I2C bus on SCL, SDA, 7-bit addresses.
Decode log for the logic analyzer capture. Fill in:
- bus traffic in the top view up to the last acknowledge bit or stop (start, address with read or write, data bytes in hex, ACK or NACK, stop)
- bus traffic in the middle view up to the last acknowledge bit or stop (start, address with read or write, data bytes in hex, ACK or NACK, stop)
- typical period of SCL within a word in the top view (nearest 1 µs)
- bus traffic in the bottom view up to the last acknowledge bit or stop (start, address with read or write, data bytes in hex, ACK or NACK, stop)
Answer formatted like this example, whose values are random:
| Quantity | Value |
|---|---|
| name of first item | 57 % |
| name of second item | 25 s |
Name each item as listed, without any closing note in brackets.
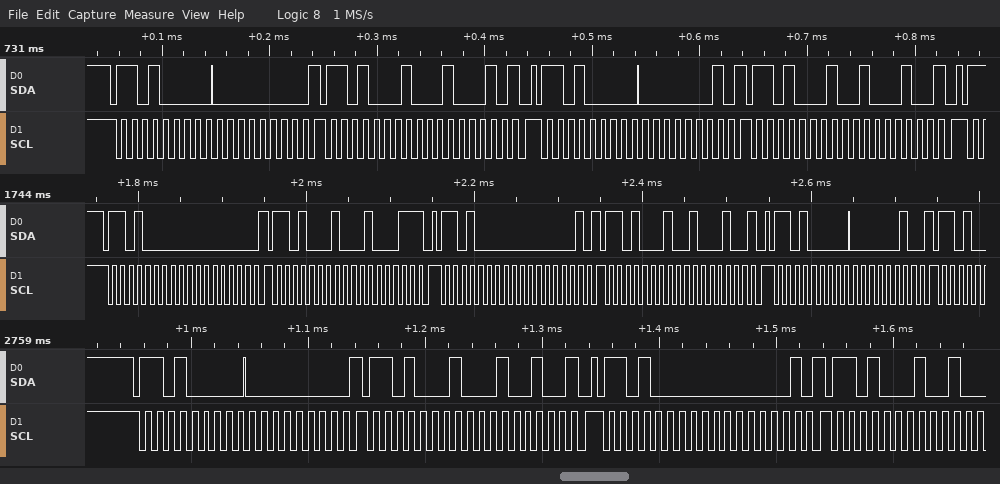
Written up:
| Quantity | Value |
|---|---|
| bus traffic in the top view up to the last acknowledge bit or stop | start, address 68 write ACK, 00 ACK, repeated start, address 68 read ACK, 22 NACK, stop, start, address 68 write ACK, 01 ACK, repeated start, address 68 read ACK, 44 NACK, stop |
| bus traffic in the middle view up to the last acknowledge bit or stop | start, address 68 write ACK, 00 ACK, repeated start, address 68 read ACK, 23 NACK, stop, start, address 68 write ACK, 01 ACK, repeated start, address 68 read ACK, 44 NACK, stop, start, address 68 write ACK, 02 ACK |
| typical period of SCL within a word in the top view | 10 µs |
| bus traffic in the bottom view up to the last acknowledge bit or stop | start, address 68 write ACK, 00 ACK, repeated start, address 68 read ACK, 24 NACK, stop, start, address 68 write ACK, 01 ACK, repeated start, address 68 read ACK |
